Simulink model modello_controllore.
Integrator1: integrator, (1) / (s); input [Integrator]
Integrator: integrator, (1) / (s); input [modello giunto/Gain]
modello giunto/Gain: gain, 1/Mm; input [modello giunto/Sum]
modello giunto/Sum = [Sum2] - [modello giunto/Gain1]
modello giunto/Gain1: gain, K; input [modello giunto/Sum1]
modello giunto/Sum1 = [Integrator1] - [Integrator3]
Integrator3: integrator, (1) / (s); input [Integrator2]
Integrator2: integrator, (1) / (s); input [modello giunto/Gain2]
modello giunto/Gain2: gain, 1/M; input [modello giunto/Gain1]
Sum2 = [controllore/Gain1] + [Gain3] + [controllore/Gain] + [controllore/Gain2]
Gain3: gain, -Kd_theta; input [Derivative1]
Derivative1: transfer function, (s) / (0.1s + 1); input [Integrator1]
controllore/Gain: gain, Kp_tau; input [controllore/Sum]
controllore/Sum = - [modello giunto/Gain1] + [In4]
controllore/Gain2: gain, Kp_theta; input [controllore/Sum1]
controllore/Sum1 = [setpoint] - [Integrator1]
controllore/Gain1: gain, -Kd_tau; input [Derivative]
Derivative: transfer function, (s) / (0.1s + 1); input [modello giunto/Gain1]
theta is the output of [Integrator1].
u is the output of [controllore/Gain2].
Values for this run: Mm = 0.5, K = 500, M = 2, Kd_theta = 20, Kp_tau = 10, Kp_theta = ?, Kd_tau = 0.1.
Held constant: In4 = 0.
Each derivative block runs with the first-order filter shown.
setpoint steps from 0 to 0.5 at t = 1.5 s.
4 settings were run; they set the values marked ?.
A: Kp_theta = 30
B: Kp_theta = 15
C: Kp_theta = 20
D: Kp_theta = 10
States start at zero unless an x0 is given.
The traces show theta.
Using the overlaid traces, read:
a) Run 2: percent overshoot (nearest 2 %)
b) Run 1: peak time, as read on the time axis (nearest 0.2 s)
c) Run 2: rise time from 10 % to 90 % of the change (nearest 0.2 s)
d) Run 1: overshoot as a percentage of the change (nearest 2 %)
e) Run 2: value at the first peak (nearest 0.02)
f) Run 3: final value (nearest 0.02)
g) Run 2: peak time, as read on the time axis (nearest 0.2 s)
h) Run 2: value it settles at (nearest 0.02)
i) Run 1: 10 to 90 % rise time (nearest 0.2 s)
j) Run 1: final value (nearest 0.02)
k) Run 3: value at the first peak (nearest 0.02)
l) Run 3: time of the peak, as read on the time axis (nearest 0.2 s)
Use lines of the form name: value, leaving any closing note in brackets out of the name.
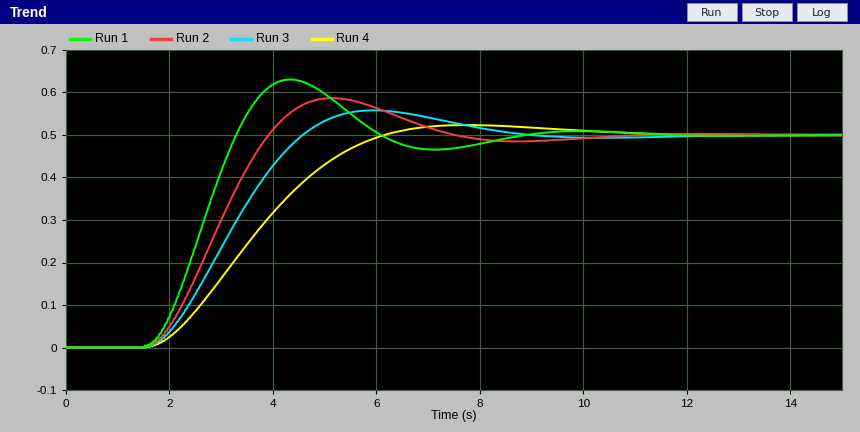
Run 2: percent overshoot: 18 %
Run 1: peak time, as read on the time axis: 4.4 s
Run 2: rise time from 10 % to 90 % of the change: 1.6 s
Run 1: overshoot as a percentage of the change: 26 %
Run 2: value at the first peak: 0.58
Run 3: final value: 0.50
Run 2: peak time, as read on the time axis: 5.2 s
Run 2: value it settles at: 0.50
Run 1: 10 to 90 % rise time: 1.2 s
Run 1: final value: 0.50
Run 3: value at the first peak: 0.56
Run 3: time of the peak, as read on the time axis: 6.0 s
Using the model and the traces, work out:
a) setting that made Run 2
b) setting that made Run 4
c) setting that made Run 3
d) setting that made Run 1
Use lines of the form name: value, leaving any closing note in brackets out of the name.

setting that made Run 2: C
setting that made Run 4: D
setting that made Run 3: B
setting that made Run 1: A
